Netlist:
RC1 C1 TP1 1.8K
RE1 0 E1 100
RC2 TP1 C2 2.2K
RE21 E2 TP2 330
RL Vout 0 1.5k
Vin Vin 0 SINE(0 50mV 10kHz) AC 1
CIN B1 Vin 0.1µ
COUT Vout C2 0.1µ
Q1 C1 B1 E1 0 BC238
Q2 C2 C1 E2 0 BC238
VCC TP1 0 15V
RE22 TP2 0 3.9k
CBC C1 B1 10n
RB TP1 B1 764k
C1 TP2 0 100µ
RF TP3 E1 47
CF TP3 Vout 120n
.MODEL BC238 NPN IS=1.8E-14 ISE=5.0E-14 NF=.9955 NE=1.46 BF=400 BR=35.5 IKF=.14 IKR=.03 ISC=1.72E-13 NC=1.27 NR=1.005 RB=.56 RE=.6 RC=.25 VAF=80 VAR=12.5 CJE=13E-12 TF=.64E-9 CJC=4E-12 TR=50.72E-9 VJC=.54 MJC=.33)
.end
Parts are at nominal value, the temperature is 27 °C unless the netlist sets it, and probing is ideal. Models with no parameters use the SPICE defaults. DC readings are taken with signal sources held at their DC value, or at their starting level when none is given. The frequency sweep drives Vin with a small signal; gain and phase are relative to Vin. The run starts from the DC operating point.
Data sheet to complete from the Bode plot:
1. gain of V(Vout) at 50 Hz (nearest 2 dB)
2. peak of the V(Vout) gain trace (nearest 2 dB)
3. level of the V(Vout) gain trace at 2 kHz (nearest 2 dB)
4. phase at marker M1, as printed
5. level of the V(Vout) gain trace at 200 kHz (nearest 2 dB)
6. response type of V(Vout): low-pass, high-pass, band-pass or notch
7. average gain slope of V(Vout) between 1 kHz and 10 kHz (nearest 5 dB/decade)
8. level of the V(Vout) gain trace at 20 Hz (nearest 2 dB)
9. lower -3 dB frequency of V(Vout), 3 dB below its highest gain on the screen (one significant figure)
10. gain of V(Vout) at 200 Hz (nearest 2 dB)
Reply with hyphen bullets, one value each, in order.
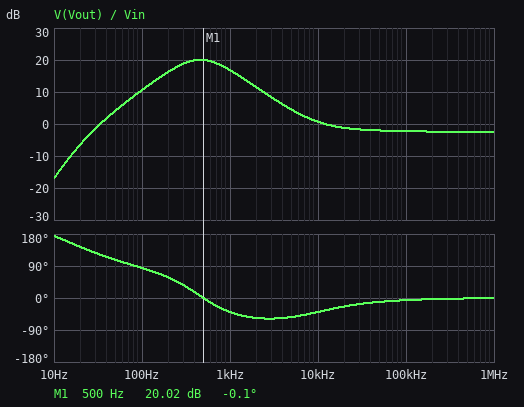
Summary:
- 4 dB
- 20 dB
- 12 dB
- -0.1 deg
- -2 dB
- band-pass
- -15 dB/decade
- -6 dB
- 200 Hz
- 16 dB
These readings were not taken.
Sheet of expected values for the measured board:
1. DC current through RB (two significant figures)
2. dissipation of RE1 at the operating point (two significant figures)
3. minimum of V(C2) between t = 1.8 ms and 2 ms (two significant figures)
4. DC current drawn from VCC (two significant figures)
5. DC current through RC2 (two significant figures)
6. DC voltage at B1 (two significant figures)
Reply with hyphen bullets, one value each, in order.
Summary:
- 18 µA
- 3.1 mW
- 13 V
- 6.6 mA
- 1.0 mA
- 1.2 V
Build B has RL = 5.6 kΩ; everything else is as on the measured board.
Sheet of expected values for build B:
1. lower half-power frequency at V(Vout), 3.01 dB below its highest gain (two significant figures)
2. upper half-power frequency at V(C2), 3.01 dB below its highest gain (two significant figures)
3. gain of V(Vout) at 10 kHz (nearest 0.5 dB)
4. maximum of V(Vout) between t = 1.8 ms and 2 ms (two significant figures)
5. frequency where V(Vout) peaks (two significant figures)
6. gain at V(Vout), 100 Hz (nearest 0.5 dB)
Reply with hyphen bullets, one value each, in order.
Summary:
- 97 Hz
- 490 Hz
- 1.0 dB
- 51 mV
- 240 Hz
- 20.5 dB
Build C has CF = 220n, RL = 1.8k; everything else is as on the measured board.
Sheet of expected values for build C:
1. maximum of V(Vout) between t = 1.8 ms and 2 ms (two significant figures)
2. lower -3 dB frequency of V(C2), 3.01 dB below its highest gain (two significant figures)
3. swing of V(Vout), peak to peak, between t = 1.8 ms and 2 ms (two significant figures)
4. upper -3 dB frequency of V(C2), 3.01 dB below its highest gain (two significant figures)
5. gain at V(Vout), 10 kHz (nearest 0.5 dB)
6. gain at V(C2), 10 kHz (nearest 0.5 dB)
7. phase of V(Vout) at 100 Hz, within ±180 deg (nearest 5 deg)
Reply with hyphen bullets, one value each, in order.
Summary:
- 46 mV
- 24 Hz
- 96 mV
- 470 Hz
- -0.5 dB
- 3.5 dB
- 75 deg
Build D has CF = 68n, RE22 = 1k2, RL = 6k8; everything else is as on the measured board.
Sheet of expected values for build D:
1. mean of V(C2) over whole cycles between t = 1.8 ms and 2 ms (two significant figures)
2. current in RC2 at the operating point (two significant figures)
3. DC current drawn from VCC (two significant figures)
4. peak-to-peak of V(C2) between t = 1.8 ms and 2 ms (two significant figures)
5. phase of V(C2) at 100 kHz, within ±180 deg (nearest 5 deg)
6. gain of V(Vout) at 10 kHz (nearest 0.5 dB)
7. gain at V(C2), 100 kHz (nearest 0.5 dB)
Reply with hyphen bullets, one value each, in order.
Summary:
- 8.8 V
- 2.8 mA
- 8.4 mA
- 230 mV
- -10 deg
- 3.5 dB
- -3.5 dB
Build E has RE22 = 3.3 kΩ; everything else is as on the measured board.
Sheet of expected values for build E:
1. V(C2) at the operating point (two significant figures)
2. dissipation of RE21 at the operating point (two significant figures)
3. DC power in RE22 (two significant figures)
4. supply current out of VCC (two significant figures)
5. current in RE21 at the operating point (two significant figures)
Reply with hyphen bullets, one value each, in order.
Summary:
- 12 V
- 480 µW
- 4.8 mW
- 6.8 mA
- 1.2 mA
